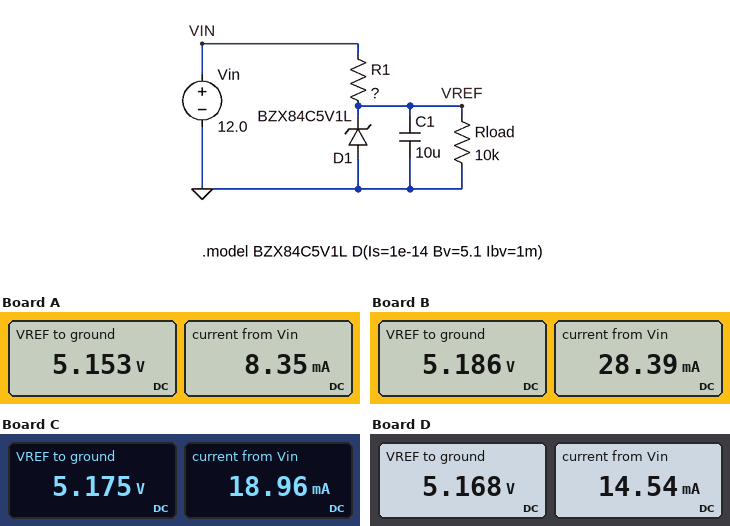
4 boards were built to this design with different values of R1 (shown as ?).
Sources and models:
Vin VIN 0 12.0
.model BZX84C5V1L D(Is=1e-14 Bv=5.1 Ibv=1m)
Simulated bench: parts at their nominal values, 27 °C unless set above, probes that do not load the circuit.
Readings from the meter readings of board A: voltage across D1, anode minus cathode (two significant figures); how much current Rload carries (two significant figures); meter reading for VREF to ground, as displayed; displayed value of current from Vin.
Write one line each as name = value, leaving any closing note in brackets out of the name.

voltage across D1, anode minus cathode = -5.2 V
how much current Rload carries = 520 µA
meter reading for VREF to ground, as displayed = 5.153 V
displayed value of current from Vin = 8.35 mA
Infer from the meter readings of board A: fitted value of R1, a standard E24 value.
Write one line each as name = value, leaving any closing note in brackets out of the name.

fitted value of R1, a standard E24 value = 820 Ω
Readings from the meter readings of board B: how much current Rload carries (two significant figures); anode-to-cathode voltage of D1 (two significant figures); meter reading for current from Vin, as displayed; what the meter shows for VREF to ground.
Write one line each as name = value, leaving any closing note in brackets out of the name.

how much current Rload carries = 520 µA
anode-to-cathode voltage of D1 = -5.2 V
meter reading for current from Vin, as displayed = 28.39 mA
what the meter shows for VREF to ground = 5.186 V
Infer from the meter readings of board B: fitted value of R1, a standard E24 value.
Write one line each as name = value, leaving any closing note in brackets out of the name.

fitted value of R1, a standard E24 value = 240 Ω
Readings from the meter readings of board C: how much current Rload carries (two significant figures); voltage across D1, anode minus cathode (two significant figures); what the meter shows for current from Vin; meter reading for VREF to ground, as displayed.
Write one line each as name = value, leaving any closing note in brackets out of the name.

how much current Rload carries = 520 µA
voltage across D1, anode minus cathode = -5.2 V
what the meter shows for current from Vin = 18.96 mA
meter reading for VREF to ground, as displayed = 5.175 V
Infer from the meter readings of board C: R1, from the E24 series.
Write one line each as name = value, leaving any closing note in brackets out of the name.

R1, from the E24 series = 360 Ω
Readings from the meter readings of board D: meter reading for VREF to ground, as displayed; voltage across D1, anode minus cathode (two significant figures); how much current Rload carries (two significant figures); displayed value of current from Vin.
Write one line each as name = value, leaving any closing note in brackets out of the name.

meter reading for VREF to ground, as displayed = 5.168 V
voltage across D1, anode minus cathode = -5.2 V
how much current Rload carries = 520 µA
displayed value of current from Vin = 14.54 mA
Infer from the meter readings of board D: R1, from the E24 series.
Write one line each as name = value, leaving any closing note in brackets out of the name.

R1, from the E24 series = 470 Ω
